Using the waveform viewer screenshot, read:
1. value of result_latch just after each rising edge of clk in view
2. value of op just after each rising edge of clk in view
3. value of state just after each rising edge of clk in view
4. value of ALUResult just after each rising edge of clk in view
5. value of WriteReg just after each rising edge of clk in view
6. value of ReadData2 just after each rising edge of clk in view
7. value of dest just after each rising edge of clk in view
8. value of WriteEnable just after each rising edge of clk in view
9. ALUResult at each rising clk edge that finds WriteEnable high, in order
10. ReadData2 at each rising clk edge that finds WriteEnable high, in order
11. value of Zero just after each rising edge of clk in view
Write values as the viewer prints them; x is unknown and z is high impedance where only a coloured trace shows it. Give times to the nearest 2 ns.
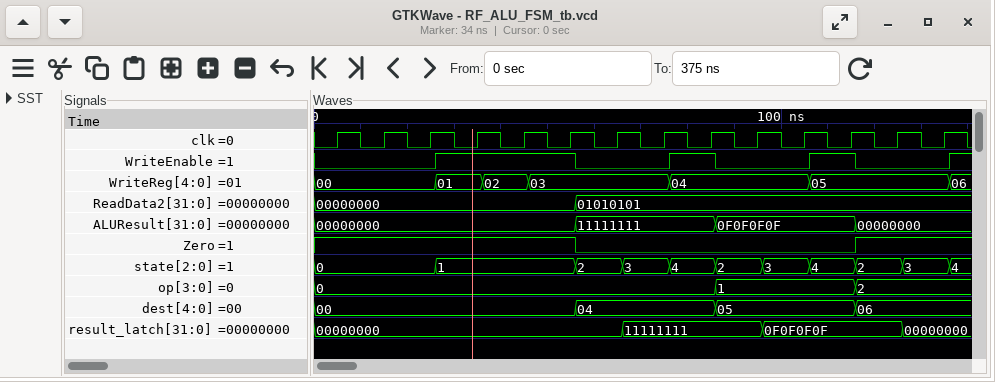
00000000, 00000000, 00000000, 00000000, 00000000, 00000000, 00000000, 11111111, 11111111, 11111111, 0F0F0F0F, 0F0F0F0F, 0F0F0F0F, 00000000
0, 0, 0, 0, 0, 0, 0, 0, 0, 1, 1, 1, 2, 2
0, 0, 0, 1, 1, 1, 2, 3, 4, 2, 3, 4, 2, 3
00000000, 00000000, 00000000, 00000000, 00000000, 00000000, 11111111, 11111111, 11111111, 0F0F0F0F, 0F0F0F0F, 0F0F0F0F, 00000000, 00000000
00, 00, 00, 01, 02, 03, 03, 03, 04, 04, 04, 05, 05, 05
00000000, 00000000, 00000000, 00000000, 00000000, 00000000, 01010101, 01010101, 01010101, 01010101, 01010101, 01010101, 01010101, 01010101
00, 00, 00, 00, 00, 00, 04, 04, 04, 05, 05, 05, 06, 06
0 0 0 1 1 1 0 0 1 0 0 1 0 0
00000000, 00000000, 00000000, 11111111, 0F0F0F0F
00000000, 00000000, 00000000, 01010101, 01010101
1 1 1 1 1 1 0 0 0 0 0 0 1 1
